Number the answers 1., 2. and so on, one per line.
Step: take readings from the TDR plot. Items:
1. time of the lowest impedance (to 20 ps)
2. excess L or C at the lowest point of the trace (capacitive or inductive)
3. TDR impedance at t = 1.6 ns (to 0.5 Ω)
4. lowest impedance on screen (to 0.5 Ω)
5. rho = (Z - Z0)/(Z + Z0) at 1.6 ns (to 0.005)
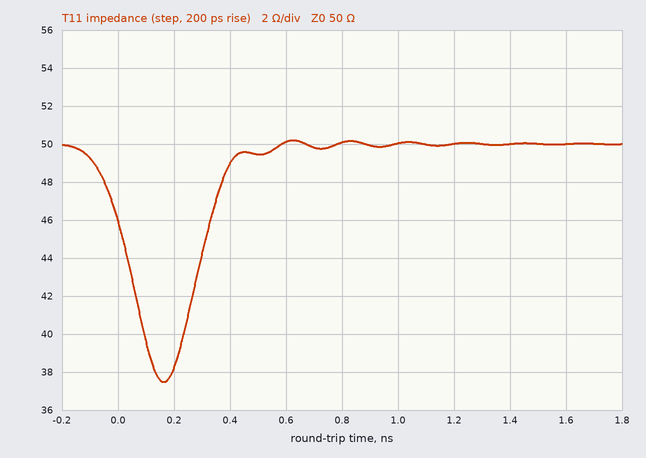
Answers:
1. 160 ps
2. capacitive
3. 50.0 Ω
4. 37.5 Ω
5. 0.000
